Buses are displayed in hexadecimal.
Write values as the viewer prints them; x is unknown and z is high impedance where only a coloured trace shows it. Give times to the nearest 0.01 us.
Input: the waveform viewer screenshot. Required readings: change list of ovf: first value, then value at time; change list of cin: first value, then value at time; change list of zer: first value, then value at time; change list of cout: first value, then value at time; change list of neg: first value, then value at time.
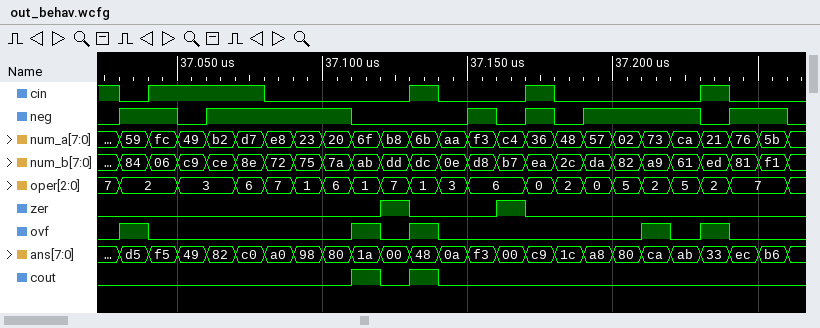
0, 1 at 37.03 us, 0 at 37.04 us, 1 at 37.11 us, 0 at 37.12 us, 1 at 37.13 us, 0 at 37.14 us, 1 at 37.21 us, 0 at 37.22 us, 1 at 37.23 us, 0 at 37.24 us
1, 0 at 37.03 us, 1 at 37.04 us, 0 at 37.08 us, 1 at 37.13 us, 0 at 37.14 us, 1 at 37.17 us, 0 at 37.18 us, 1 at 37.23 us, 0 at 37.24 us
0, 1 at 37.12 us, 0 at 37.13 us, 1 at 37.16 us, 0 at 37.17 us
0, 1 at 37.11 us, 0 at 37.12 us, 1 at 37.13 us, 0 at 37.14 us
0, 1 at 37.03 us, 0 at 37.05 us, 1 at 37.06 us, 0 at 37.11 us, 1 at 37.15 us, 0 at 37.16 us, 1 at 37.17 us, 0 at 37.18 us, 1 at 37.19 us, 0 at 37.23 us, 1 at 37.24 us, 0 at 37.26 us
